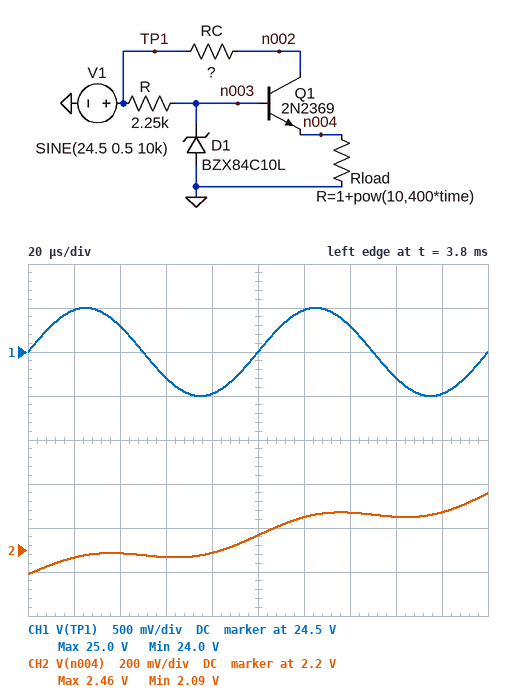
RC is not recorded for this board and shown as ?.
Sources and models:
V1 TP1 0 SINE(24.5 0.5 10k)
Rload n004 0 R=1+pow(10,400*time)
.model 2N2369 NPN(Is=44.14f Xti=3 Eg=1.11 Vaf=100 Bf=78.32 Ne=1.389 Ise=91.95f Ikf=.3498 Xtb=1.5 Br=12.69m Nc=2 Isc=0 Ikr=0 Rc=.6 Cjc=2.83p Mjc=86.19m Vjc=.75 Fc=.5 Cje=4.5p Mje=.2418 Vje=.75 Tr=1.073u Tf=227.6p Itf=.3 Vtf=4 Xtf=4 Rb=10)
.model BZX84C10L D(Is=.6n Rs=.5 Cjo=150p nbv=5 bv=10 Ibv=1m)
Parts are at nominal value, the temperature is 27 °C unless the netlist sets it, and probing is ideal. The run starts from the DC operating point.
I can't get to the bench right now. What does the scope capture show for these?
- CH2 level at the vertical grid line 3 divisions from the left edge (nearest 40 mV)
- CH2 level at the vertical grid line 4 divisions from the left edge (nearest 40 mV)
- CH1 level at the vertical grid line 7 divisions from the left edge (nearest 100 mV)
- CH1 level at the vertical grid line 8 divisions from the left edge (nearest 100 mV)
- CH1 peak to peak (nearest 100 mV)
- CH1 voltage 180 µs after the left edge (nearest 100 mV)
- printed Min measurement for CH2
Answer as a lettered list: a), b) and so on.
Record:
a) 2.16 V
b) 2.20 V
c) 24.8 V
d) 24.2 V
e) 1.0 V
f) 24.0 V
g) 2.09 V
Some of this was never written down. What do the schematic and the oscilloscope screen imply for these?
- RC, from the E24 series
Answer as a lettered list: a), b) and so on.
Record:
a) 430 Ω
